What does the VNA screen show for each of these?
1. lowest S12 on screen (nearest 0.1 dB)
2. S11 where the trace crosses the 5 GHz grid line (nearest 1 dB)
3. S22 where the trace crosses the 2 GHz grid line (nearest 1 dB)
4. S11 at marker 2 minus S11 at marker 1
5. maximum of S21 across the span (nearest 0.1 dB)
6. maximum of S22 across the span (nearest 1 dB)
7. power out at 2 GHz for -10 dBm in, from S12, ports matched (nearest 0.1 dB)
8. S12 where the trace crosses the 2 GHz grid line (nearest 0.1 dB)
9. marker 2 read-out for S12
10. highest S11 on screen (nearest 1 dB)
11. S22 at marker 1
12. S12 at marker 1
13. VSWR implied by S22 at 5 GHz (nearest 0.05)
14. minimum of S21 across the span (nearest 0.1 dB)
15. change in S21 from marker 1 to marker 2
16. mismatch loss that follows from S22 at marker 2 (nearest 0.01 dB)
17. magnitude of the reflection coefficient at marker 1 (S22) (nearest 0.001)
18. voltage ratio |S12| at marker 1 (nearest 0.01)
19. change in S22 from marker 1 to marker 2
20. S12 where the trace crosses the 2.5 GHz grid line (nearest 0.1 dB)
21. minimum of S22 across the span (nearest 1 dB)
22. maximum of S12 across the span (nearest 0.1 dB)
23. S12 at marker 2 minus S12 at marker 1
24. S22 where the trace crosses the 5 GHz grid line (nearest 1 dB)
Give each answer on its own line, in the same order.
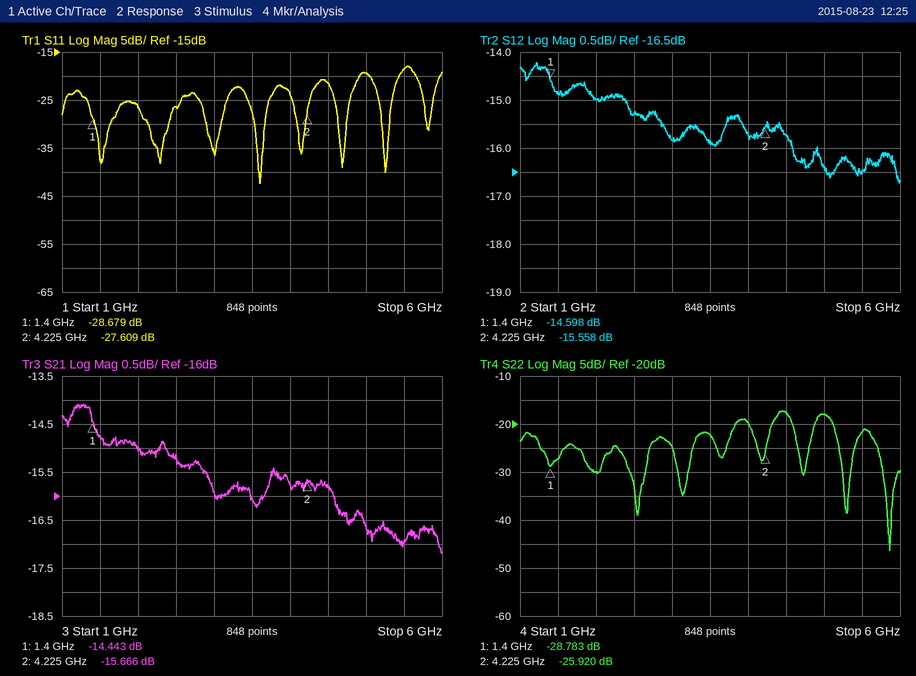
-16.7 dB
-19 dB
-30 dB
1.070 dB
-14.1 dB
-17 dB
-25.0 dBm
-15.0 dB
-15.558 dB
-18 dB
-28.783 dB
-14.598 dB
1.30
-17.2 dB
-1.223 dB
0.01 dB
0.036
0.19
2.863 dB
-15.3 dB
-46 dB
-14.2 dB
-0.960 dB
-18 dB
